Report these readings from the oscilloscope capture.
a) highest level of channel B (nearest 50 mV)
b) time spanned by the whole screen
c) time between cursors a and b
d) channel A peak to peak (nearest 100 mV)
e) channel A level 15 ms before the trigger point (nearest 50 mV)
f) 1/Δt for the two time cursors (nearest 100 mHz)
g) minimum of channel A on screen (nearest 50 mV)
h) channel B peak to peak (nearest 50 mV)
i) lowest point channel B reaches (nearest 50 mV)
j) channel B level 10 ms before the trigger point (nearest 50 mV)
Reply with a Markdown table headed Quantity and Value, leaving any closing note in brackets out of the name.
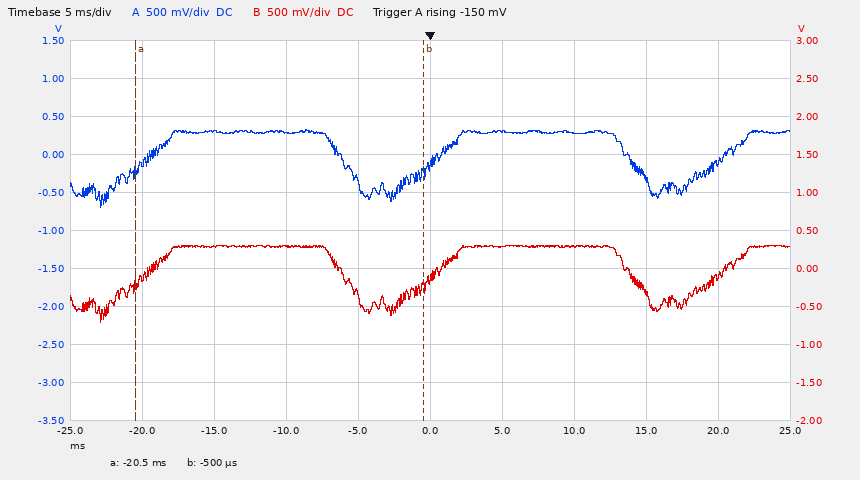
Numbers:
| Quantity | Value |
|---|---|
| highest level of channel B | 300 mV |
| time spanned by the whole screen | 50 ms |
| time between cursors a and b | 20.0 ms |
| channel A peak to peak | 1.00 V |
| channel A level 15 ms before the trigger point | 300 mV |
| 1/Δt for the two time cursors | 50.0 Hz |
| minimum of channel A on screen | -700 mV |
| channel B peak to peak | 1.00 V |
| lowest point channel B reaches | -700 mV |
| channel B level 10 ms before the trigger point | 300 mV |
